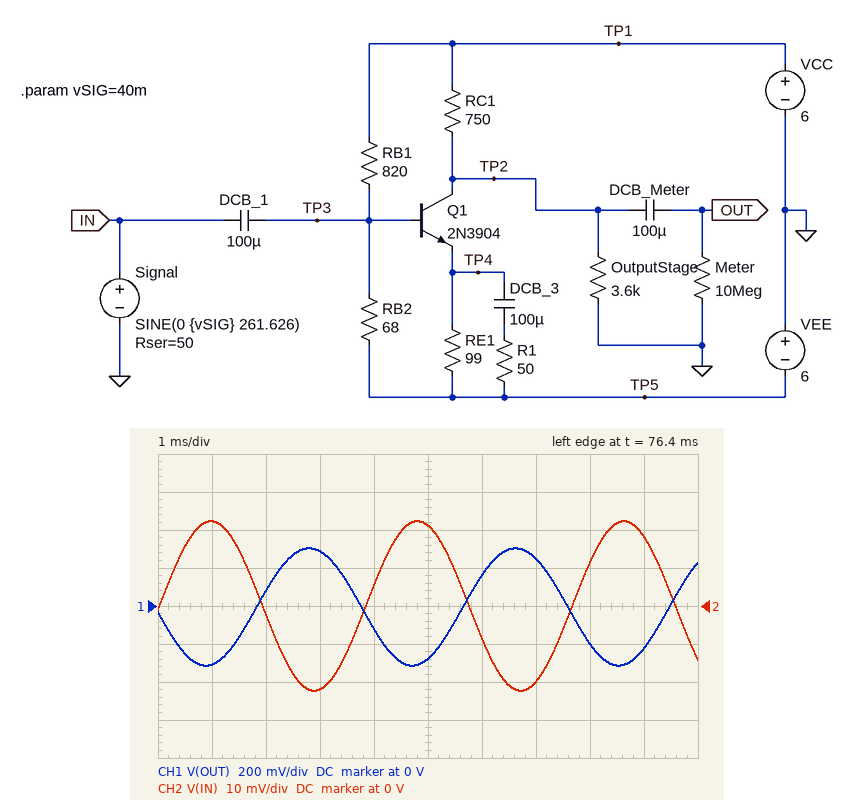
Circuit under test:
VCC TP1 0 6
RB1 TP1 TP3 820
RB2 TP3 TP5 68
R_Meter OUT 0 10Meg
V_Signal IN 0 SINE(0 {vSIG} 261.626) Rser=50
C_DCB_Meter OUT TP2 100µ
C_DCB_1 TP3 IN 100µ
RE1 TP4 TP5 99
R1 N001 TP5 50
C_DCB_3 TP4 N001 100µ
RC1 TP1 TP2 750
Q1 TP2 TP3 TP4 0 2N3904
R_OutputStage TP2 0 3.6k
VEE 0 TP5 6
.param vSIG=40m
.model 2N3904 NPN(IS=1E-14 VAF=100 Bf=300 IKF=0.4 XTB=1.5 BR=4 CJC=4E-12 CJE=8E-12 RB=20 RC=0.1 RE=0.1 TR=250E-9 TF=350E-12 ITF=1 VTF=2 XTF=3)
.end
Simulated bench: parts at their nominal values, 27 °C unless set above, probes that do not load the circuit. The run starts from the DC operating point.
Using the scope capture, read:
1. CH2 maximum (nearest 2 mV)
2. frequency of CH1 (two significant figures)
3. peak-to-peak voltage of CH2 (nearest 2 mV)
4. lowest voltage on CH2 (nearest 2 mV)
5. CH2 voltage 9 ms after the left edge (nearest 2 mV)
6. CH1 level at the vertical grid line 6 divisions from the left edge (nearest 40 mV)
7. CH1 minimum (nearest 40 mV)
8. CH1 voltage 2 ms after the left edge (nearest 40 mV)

22 mV
260 Hz
44 mV
-22 mV
18 mV
160 mV
-320 mV
80 mV
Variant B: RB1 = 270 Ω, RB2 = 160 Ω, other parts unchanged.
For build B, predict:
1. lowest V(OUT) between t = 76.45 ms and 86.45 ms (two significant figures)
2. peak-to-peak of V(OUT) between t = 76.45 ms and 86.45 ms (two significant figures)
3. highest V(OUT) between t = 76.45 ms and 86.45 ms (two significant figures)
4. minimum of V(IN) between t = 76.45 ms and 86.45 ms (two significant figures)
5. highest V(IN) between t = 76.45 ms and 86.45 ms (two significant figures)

-9.6 mV
19 mV
9.6 mV
-17 mV
17 mV
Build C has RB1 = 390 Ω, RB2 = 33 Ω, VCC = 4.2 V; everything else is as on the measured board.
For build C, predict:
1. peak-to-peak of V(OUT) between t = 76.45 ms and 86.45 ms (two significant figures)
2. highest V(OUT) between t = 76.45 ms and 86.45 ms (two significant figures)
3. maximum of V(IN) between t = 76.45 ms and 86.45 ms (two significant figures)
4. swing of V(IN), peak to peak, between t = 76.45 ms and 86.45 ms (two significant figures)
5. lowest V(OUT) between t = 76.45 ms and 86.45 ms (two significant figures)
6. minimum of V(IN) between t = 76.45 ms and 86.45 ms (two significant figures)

350 mV
170 mV
15 mV
31 mV
-180 mV
-15 mV
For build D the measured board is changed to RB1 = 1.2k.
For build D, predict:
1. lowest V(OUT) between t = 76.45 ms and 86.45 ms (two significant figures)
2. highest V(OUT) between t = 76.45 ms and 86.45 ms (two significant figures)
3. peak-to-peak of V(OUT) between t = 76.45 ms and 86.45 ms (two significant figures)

-120 mV
83 mV
210 mV
